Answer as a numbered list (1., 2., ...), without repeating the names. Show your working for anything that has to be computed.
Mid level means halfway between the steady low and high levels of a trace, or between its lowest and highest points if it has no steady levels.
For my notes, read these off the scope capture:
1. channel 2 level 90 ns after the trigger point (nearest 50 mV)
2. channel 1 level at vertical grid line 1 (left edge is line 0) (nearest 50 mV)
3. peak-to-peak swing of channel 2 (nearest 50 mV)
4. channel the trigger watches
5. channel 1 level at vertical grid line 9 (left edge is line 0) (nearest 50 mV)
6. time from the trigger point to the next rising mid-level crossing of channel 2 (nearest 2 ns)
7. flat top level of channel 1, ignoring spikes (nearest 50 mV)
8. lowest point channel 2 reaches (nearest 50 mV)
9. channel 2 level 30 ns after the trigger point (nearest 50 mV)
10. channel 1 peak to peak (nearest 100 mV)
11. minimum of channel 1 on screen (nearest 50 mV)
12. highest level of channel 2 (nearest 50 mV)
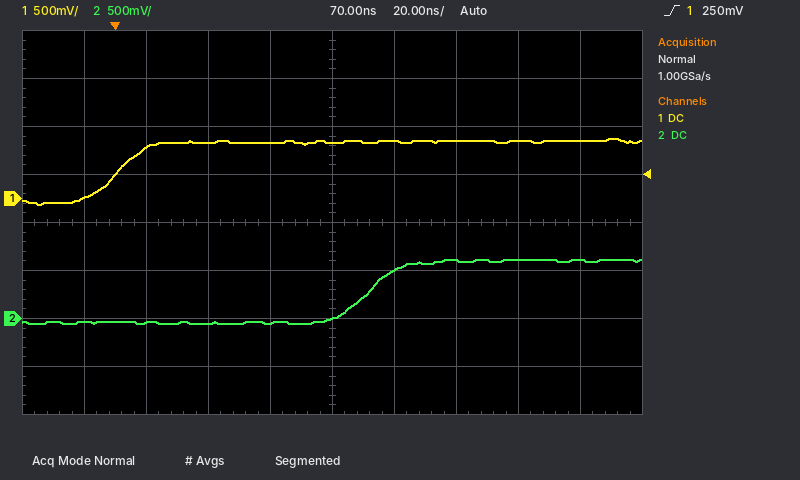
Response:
1. 500 mV
2. 0 mV
3. 600 mV − (-50 mV) = 650 mV
4. channel 1
5. 600 mV
6. 82 ns
7. 600 mV
8. -50 mV
9. -50 mV
10. 700 mV
11. -50 mV
12. 600 mV
